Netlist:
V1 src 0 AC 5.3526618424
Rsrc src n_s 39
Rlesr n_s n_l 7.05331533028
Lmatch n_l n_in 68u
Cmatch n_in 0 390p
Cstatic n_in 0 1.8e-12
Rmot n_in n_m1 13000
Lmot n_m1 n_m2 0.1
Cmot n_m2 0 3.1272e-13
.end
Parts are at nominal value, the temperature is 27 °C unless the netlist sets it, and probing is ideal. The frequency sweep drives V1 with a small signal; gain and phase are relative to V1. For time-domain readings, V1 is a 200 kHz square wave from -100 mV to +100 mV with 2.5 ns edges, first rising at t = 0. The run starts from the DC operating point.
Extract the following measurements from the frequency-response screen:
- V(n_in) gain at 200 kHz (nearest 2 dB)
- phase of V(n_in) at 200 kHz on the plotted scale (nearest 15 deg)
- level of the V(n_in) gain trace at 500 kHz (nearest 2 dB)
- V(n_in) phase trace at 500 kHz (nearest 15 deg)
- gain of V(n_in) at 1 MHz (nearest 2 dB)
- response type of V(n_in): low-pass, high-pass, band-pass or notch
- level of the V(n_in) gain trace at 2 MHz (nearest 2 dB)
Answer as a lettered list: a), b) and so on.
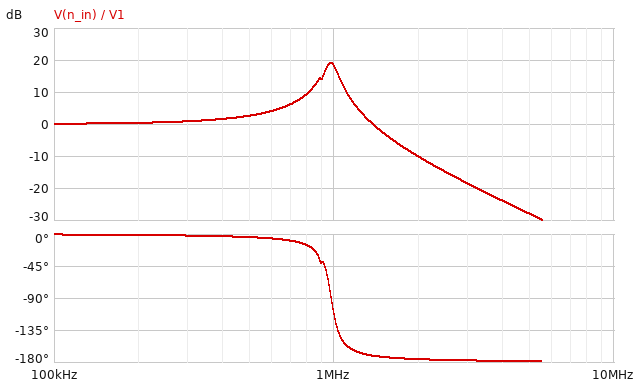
a) 0 dB
b) 0 deg
c) 2 dB
d) 0 deg
e) 18 dB
f) low-pass
g) -10 dB
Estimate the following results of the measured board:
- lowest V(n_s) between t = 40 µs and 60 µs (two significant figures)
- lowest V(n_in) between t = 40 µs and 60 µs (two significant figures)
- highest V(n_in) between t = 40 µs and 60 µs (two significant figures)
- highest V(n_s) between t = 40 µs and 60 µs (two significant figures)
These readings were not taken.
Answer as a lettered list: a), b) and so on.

a) -120 mV
b) -360 mV
c) 360 mV
d) 120 mV
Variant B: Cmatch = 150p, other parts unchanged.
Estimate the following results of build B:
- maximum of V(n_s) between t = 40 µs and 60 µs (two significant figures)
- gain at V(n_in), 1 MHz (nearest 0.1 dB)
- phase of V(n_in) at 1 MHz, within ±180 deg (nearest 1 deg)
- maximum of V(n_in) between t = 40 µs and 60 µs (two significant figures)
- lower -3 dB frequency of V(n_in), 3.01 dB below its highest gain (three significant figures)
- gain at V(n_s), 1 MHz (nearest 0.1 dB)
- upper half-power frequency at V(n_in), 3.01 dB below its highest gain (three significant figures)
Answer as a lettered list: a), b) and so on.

a) 110 mV
b) 4.5 dB
c) -4 deg
d) 230 mV
e) 1.51 MHz
f) 0 dB
g) 1.62 MHz
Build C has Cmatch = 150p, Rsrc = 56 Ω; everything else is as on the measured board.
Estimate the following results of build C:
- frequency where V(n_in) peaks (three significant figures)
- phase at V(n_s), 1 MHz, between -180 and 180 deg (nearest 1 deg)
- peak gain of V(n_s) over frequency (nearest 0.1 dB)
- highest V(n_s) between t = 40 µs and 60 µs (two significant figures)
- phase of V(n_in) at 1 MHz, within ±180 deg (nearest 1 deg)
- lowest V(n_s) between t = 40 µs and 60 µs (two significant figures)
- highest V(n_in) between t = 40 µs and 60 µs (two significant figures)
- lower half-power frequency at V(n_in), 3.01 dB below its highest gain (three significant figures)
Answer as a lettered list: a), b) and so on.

a) 1.56 MHz
b) -5 deg
c) 0 dB
d) 110 mV
e) -6 deg
f) -110 mV
g) 240 mV
h) 1.49 MHz
